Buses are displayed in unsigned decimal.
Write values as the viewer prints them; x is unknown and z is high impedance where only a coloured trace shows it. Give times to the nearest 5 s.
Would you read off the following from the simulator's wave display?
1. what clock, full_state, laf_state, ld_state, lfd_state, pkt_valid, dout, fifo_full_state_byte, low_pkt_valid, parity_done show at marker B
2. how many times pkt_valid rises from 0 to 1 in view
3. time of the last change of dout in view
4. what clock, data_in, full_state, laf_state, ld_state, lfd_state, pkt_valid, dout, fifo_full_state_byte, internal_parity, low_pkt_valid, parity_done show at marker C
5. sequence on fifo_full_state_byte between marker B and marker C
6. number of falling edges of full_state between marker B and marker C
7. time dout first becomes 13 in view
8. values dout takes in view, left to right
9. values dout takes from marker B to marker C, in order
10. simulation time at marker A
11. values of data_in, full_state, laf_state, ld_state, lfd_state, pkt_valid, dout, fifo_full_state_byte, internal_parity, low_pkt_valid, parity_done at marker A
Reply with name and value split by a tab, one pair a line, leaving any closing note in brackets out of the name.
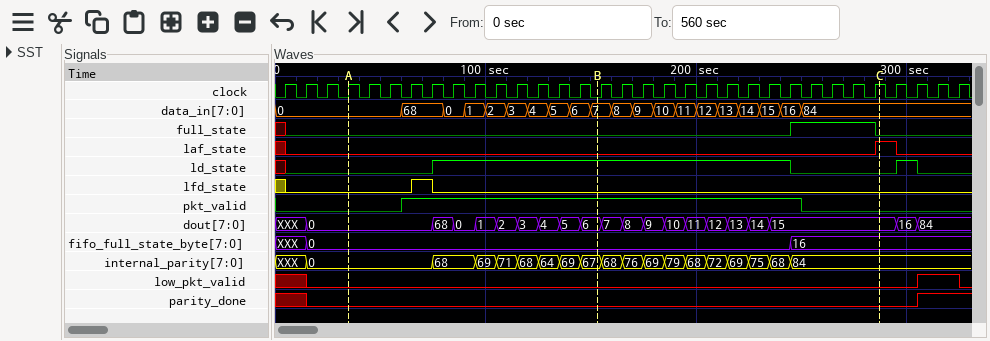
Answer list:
what clock, full_state, laf_state, ld_state, lfd_state, pkt_valid, dout, fifo_full_state_byte, low_pkt_valid, parity_done show at marker B	clock=0, full_state=0, laf_state=0, ld_state=1, lfd_state=0, pkt_valid=1, dout=6, fifo_full_state_byte=0, low_pkt_valid=0, parity_done=0
how many times pkt_valid rises from 0 to 1 in view	1
time of the last change of dout in view	305 s
what clock, data_in, full_state, laf_state, ld_state, lfd_state, pkt_valid, dout, fifo_full_state_byte, internal_parity, low_pkt_valid, parity_done show at marker C	clock=1, data_in=84, full_state=0, laf_state=1, ld_state=0, lfd_state=0, pkt_valid=0, dout=15, fifo_full_state_byte=16, internal_parity=84, low_pkt_valid=0, parity_done=0
sequence on fifo_full_state_byte between marker B and marker C	0, 16
number of falling edges of full_state between marker B and marker C	1
time dout first becomes 13 in view	215 s
values dout takes in view, left to right	XXX, 0, 68, 0, 1, 2, 3, 4, 5, 6, 7, 8, 9, 10, 11, 12, 13, 14, 15, 16, 84
values dout takes from marker B to marker C, in order	6, 7, 8, 9, 10, 11, 12, 13, 14, 15
simulation time at marker A	35 s
values of data_in, full_state, laf_state, ld_state, lfd_state, pkt_valid, dout, fifo_full_state_byte, internal_parity, low_pkt_valid, parity_done at marker A	data_in=0, full_state=0, laf_state=0, ld_state=0, lfd_state=0, pkt_valid=0, dout=0, fifo_full_state_byte=0, internal_parity=0, low_pkt_valid=0, parity_done=0
